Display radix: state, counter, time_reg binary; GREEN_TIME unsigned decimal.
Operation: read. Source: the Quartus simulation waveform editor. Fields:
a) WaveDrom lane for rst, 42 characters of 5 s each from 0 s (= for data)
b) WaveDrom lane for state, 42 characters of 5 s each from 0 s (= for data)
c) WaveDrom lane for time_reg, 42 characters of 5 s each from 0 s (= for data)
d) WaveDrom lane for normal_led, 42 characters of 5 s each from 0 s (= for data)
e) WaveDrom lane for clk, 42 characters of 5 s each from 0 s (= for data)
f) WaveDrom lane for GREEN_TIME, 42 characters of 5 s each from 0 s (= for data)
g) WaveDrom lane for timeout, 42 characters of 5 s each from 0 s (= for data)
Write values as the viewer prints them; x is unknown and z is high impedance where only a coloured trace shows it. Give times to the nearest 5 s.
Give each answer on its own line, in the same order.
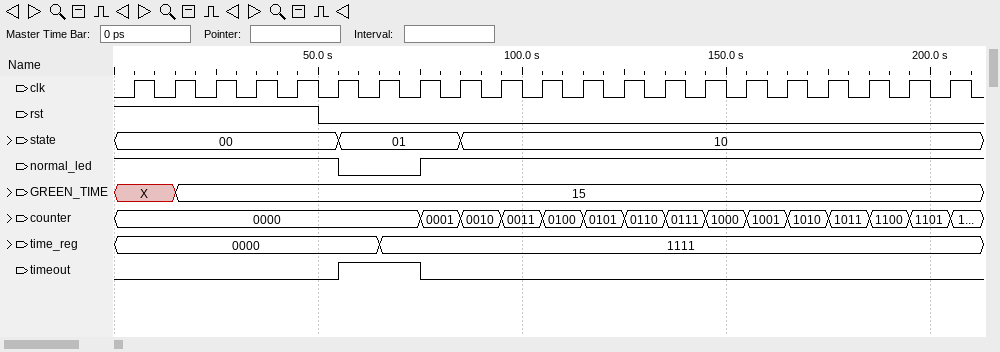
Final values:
{name: 'rst', wave: '1.........0...............................'}
{name: 'state', wave: '=..........=.....=........................', data: '00 01 10'}
{name: 'time_reg', wave: '=............=............................', data: '0000 1111'}
{name: 'normal_led', wave: '1..........0...1..........................'}
{name: 'clk', wave: '010101010101010101010101010101010101010101'}
{name: 'GREEN_TIME', wave: 'x..=......................................', data: '15'}
{name: 'timeout', wave: '0..........1...0..........................'}
